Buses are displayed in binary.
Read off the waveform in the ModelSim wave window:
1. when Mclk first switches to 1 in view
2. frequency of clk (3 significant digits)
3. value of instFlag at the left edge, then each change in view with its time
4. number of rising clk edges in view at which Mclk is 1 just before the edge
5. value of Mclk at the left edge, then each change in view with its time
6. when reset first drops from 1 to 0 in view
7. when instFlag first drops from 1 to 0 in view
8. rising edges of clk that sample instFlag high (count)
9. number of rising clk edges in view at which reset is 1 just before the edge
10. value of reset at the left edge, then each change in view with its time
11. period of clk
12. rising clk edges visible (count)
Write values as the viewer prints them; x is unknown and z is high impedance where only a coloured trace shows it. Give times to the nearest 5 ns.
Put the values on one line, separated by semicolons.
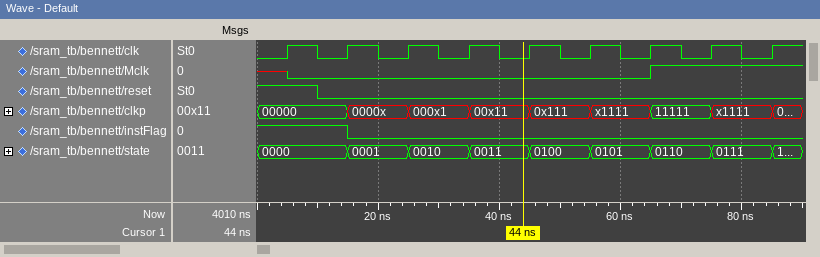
65 ns; 100 MHz; 1, 0 at 15 ns; 2; x, 0 at 5 ns, 1 at 65 ns; 10 ns; 15 ns; 2; 1; 1, 0 at 10 ns; 10 ns; 9
